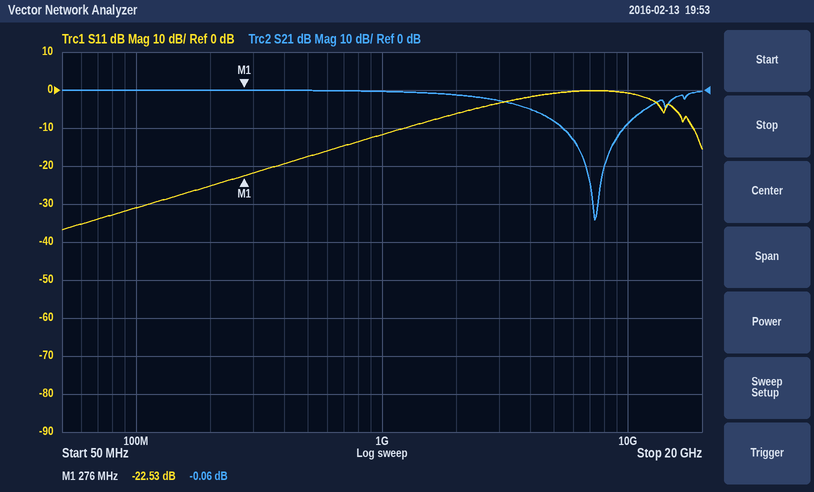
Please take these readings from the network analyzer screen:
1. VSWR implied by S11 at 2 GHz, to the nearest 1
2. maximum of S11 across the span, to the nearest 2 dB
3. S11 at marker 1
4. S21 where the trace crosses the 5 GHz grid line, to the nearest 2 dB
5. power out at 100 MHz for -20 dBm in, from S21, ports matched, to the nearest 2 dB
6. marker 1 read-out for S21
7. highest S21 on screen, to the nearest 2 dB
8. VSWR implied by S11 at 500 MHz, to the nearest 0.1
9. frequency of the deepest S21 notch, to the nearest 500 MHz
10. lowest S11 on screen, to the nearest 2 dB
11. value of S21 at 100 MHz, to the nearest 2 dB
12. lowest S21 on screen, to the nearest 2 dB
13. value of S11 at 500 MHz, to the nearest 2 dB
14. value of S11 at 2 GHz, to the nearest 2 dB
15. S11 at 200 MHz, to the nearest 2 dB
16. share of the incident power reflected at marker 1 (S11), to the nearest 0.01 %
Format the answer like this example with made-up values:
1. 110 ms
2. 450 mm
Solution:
1. 3
2. 0 dB
3. -22.53 dB
4. -8 dB
5. -20 dBm
6. -0.06 dB
7. 0 dB
8. 1.3
9. 7.5 GHz
10. -36 dB
11. 0 dB
12. -34 dB
13. -18 dB
14. -6 dB
15. -26 dB
16. 0.56 %
